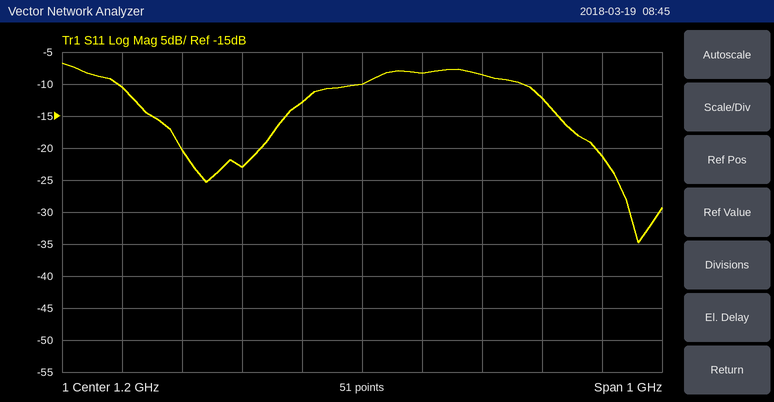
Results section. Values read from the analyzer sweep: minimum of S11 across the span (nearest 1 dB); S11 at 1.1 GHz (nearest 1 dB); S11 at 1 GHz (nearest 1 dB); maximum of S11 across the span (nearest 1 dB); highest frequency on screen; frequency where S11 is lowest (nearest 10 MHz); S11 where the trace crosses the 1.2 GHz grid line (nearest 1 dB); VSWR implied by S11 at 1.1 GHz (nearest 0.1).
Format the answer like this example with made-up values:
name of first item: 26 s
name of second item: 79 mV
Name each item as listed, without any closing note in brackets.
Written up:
minimum of S11 across the span: -35 dB
S11 at 1.1 GHz: -13 dB
S11 at 1 GHz: -23 dB
maximum of S11 across the span: -7 dB
highest frequency on screen: 1.7 GHz
frequency where S11 is lowest: 1.66 GHz
S11 where the trace crosses the 1.2 GHz grid line: -10 dB
VSWR implied by S11 at 1.1 GHz: 1.6
